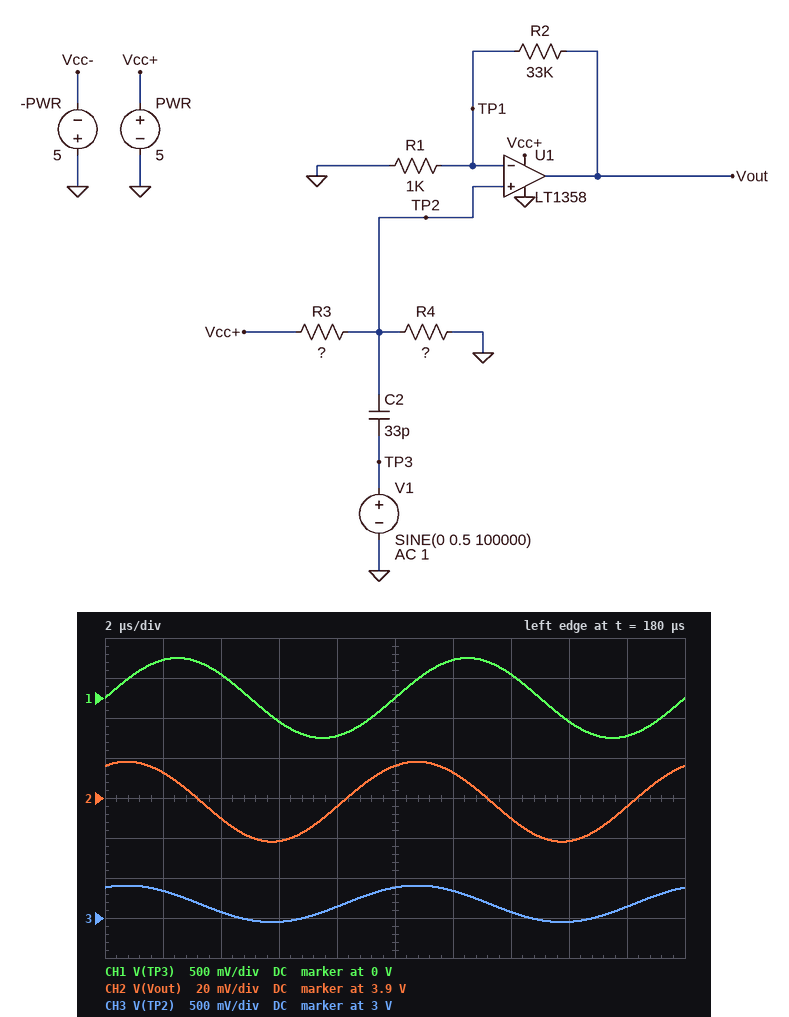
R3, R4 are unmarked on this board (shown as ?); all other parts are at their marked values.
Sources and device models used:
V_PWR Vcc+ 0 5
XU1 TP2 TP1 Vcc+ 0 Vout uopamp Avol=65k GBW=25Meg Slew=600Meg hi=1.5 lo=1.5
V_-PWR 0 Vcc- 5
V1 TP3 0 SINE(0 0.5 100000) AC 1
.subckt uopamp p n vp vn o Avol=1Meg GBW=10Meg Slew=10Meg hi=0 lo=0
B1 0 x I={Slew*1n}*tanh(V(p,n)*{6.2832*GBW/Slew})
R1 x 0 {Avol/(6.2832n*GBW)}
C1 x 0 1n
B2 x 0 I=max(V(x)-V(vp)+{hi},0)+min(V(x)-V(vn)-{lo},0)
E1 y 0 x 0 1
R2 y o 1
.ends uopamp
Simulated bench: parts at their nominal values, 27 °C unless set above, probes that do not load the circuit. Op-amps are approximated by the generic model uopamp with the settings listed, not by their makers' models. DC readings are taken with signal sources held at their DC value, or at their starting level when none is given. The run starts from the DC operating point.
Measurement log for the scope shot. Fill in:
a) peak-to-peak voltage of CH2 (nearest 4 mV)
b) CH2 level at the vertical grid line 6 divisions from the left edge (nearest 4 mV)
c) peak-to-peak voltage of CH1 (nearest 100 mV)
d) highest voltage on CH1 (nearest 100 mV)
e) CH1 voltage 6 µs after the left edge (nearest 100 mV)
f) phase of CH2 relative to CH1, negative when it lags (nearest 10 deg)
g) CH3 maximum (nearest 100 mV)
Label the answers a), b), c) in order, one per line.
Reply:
a) 40 mV
b) 3.912 V
c) 1.0 V
d) 500 mV
e) -300 mV
f) 60 deg
g) 3.4 V
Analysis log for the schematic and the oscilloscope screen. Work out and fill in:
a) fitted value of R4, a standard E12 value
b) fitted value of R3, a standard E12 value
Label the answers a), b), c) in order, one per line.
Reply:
a) 68 kΩ
b) 39 kΩ
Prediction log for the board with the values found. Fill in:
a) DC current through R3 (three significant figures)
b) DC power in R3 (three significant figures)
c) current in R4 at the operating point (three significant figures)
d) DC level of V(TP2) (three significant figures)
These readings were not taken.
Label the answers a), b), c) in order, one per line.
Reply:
a) 46.7 µA
b) 85.2 µW
c) 46.7 µA
d) 3.18 V
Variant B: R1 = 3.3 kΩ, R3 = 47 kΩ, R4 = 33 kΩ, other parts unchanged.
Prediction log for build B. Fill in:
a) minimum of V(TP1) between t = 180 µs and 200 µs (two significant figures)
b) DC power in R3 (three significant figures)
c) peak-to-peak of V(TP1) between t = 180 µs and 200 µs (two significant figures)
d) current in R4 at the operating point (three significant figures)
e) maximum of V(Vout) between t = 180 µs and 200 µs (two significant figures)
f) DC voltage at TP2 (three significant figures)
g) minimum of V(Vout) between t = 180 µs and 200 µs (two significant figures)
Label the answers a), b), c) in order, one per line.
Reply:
a) 340 mV
b) 184 µW
c) 4.3 mV
d) 62.5 µA
e) 3.8 V
f) 2.06 V
g) 3.7 V
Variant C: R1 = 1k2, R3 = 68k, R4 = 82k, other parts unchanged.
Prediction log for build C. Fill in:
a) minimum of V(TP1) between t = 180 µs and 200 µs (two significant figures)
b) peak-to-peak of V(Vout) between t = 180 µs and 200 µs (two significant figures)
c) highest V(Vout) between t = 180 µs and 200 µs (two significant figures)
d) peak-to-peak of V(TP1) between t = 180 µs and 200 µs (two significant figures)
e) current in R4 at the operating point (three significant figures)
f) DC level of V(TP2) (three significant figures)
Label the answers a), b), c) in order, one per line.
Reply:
a) 130 mV
b) 62 mV
c) 3.9 V
d) 2.2 mV
e) 33.3 µA
f) 2.73 V
